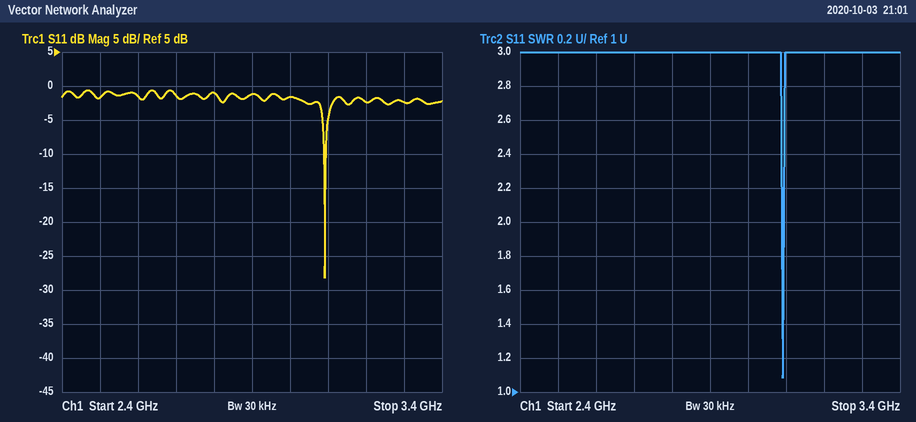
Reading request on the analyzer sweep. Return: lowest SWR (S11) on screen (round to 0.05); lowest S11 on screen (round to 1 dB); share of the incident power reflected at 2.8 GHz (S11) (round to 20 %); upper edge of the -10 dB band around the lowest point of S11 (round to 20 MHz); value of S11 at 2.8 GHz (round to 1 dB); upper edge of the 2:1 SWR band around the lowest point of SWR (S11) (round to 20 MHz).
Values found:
1.10
-28 dB
80 %
3.10 GHz
-1 dB
3.10 GHz
